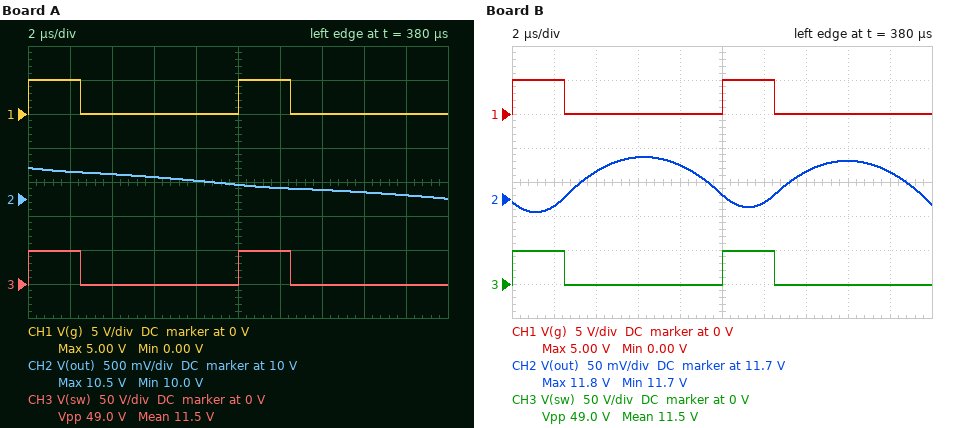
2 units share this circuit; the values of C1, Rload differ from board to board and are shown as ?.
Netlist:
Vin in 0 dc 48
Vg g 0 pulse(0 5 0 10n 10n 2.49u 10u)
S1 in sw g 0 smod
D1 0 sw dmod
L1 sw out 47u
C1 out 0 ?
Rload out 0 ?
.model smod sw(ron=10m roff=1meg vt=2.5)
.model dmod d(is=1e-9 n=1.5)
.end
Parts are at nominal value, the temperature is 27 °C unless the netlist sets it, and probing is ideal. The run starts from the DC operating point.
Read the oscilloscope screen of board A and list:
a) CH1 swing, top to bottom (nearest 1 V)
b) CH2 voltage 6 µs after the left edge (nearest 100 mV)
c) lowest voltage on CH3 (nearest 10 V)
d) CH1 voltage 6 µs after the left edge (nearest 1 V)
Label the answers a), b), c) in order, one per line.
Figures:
a) 5 V
b) 10.3 V
c) 0 V
d) 0 V
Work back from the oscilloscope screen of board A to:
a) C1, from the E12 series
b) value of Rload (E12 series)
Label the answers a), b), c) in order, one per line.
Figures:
a) 100 µF
b) 1.2 Ω
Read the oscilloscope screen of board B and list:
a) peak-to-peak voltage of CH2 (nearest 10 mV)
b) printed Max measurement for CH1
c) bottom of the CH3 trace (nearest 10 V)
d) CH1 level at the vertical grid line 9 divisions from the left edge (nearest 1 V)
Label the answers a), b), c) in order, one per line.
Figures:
a) 80 mV
b) 5.00 V
c) 0 V
d) 0 V
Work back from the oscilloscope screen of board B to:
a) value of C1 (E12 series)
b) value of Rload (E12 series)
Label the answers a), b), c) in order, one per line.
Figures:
a) 33 µF
b) 1.8 Ω
